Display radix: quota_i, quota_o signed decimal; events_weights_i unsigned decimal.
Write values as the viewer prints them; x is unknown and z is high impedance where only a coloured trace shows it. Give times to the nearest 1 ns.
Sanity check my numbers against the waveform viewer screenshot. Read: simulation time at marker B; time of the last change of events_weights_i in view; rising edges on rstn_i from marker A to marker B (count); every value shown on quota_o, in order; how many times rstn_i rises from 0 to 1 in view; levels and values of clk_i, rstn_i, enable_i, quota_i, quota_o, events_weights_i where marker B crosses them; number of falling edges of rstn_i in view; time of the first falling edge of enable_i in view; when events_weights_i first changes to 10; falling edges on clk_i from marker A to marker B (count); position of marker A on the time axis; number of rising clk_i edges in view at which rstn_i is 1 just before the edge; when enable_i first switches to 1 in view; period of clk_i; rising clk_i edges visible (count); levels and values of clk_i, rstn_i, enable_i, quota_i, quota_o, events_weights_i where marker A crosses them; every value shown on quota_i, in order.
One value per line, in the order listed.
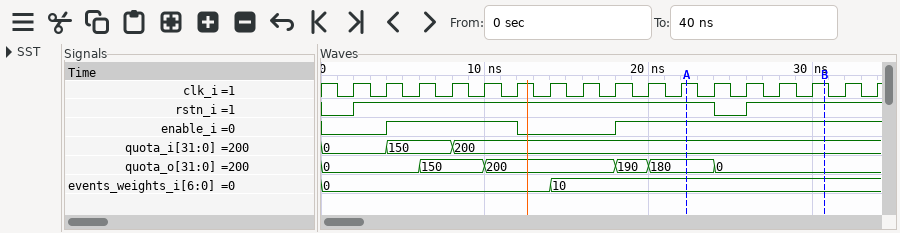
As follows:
31 ns
14 ns
1
0, 150, 200, 190, 180, 0
2
clk_i=1, rstn_i=1, enable_i=1, quota_i=200, quota_o=0, events_weights_i=10
1
12 ns
14 ns
4
22 ns
15
4 ns
2 ns
17
clk_i=1, rstn_i=1, enable_i=1, quota_i=200, quota_o=180, events_weights_i=10
0, 150, 200
